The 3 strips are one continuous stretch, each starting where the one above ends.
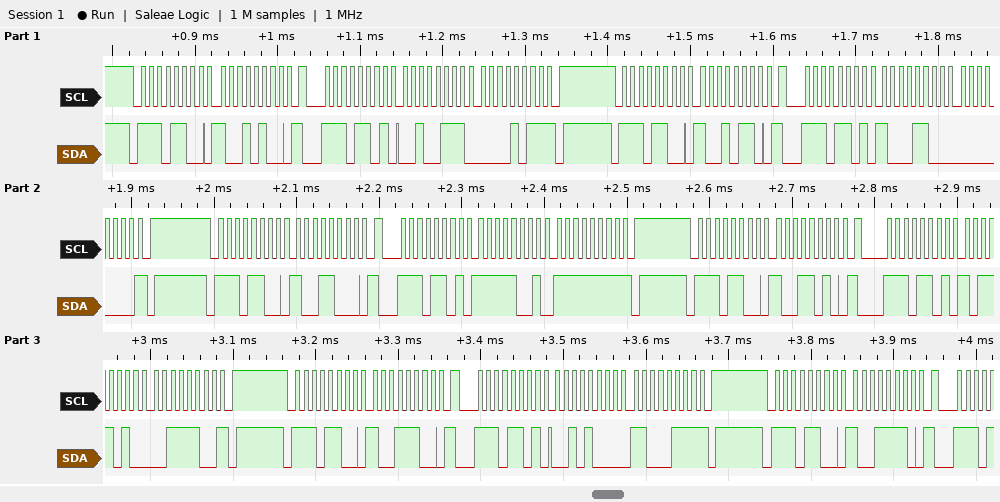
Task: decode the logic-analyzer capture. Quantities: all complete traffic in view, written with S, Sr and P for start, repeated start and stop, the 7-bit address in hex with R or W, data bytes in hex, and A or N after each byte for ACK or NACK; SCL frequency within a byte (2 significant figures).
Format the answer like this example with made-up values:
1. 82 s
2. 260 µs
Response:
1. S 76W A 94 A Sr 76R A 27 A 0B N P S 76W A 96 A Sr 76R A 8C A 00 N P S 76W A 98 A Sr 76R A F9 A FF N P S 76W A 9A A Sr 76R A BA A 3C N P S 76W A 9C A Sr 76R A 28 A C7 N P S 76W A 9E A
2. 100 kHz
